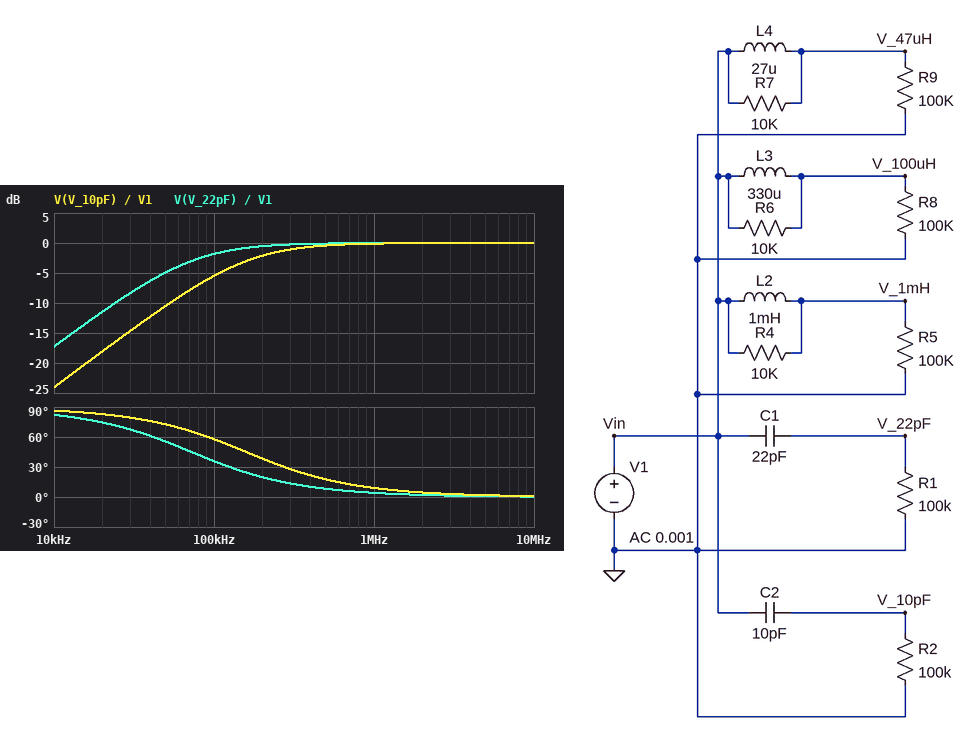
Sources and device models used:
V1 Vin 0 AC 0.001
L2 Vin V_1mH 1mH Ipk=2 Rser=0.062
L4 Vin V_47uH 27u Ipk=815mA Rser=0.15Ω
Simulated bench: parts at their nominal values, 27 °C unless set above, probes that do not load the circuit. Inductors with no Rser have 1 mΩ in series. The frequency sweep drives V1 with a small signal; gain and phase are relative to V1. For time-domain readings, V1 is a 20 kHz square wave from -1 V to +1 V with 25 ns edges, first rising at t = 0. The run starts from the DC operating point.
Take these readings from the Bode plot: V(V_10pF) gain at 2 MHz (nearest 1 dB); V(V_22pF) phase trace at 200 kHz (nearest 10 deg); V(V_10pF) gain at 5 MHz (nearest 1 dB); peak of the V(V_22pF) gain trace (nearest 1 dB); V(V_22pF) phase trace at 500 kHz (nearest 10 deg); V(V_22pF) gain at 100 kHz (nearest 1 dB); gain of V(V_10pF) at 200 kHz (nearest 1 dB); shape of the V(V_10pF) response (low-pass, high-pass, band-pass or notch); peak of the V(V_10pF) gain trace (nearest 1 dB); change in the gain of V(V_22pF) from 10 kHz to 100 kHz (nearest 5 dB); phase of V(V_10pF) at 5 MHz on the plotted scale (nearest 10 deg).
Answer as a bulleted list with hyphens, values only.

- 0 dB
- 20 deg
- 0 dB
- 0 dB
- 10 deg
- -2 dB
- -2 dB
- high-pass
- 0 dB
- 15 dB
- 0 deg
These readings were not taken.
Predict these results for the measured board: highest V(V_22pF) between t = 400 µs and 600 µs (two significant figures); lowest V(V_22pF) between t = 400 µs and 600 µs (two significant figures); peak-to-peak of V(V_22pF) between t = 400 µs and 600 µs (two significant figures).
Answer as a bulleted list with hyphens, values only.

- 2.0 V
- -2.0 V
- 4.0 V
